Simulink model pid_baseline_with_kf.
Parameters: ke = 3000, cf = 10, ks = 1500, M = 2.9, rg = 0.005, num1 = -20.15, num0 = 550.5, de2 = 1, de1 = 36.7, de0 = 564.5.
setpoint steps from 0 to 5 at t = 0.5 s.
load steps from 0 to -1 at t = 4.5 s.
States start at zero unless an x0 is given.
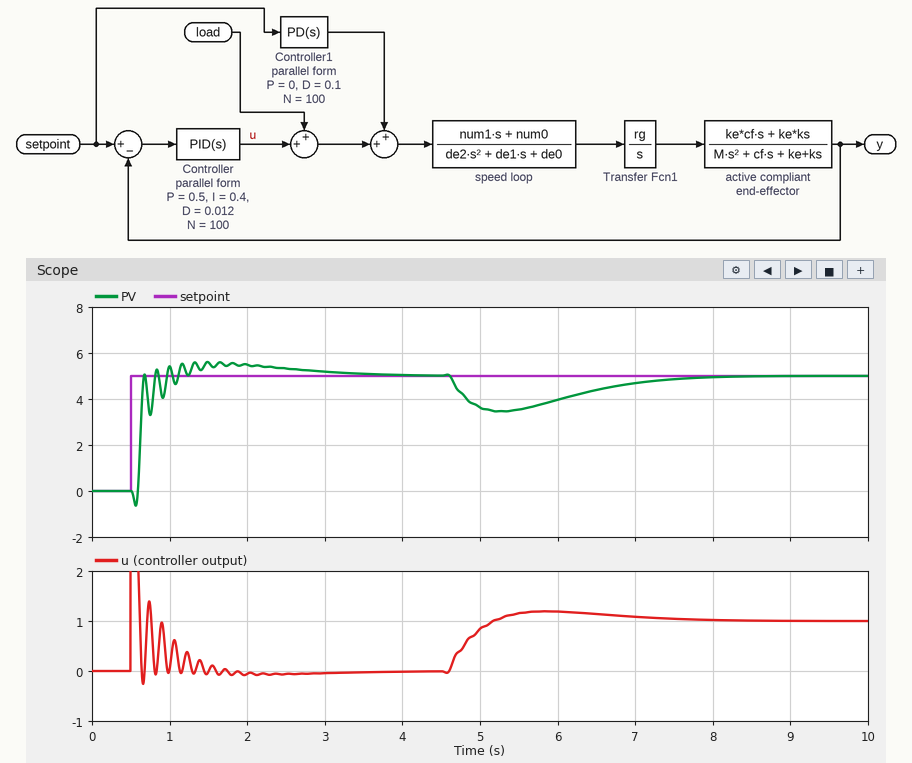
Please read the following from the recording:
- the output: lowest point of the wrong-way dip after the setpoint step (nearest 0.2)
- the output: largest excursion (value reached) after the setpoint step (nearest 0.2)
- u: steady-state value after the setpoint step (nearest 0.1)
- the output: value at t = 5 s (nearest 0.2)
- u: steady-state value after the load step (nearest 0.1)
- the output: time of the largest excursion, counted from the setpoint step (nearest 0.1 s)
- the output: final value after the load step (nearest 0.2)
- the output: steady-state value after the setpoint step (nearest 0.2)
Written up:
-0.6
5.6
0.0
3.6
1.0
1.0 s
5.0
5.0
